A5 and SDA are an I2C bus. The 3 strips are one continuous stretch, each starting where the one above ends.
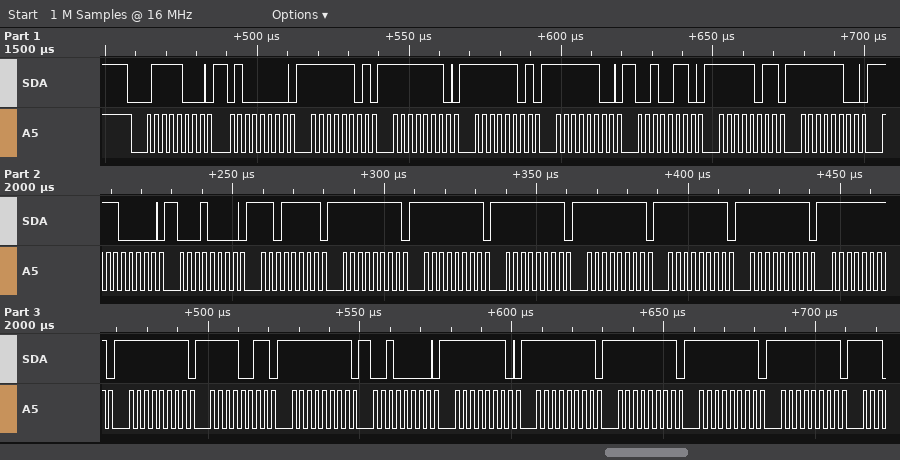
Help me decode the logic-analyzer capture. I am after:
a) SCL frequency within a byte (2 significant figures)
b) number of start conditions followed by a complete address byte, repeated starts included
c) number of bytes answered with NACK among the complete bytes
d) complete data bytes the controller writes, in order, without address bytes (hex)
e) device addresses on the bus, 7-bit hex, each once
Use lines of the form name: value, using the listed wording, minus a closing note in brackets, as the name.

SCL frequency within a byte: 400 kHz
number of start conditions followed by a complete address byte, repeated starts included: 1
number of bytes answered with NACK among the complete bytes: 0
complete data bytes the controller writes, in order, without address bytes: 40 FD FE FD FC 26 FB FC E0 10 DF FF FF FF FF FF FF FF FF F3 FF 20 FE FF FF FF FF
device addresses on the bus, 7-bit hex, each once: 0x3C
